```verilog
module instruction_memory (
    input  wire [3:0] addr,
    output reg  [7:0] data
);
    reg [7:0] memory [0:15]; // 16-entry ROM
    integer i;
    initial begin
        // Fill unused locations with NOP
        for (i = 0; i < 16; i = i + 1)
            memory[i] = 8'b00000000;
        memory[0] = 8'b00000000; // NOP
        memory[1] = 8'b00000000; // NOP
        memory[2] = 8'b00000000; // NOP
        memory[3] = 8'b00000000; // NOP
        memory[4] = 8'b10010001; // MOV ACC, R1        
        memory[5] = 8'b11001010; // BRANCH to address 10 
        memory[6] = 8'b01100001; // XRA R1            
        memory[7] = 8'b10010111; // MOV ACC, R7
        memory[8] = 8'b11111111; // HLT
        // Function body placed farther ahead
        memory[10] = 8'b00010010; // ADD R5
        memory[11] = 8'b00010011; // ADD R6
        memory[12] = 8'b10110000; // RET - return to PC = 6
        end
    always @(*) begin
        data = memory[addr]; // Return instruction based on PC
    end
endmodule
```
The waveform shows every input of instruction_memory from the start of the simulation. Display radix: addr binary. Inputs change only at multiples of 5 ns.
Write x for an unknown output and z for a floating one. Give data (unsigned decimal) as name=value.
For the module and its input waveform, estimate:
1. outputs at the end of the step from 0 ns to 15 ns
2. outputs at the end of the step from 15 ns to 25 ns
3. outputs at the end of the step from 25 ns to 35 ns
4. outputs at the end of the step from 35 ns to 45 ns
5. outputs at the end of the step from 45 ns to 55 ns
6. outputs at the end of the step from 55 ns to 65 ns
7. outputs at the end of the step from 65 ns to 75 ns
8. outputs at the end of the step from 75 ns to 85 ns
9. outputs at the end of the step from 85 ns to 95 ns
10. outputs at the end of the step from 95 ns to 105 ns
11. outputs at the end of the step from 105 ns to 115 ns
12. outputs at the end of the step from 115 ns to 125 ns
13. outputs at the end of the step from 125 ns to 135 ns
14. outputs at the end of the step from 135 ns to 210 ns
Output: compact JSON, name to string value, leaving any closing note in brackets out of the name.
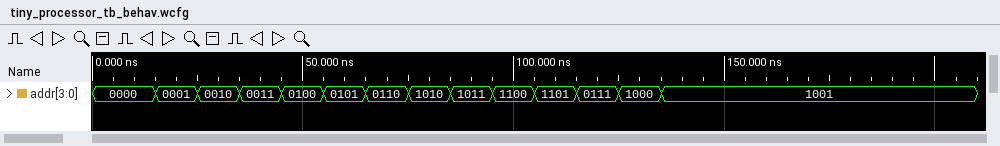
{"outputs at the end of the step from 0 ns to 15 ns": "data=0", "outputs at the end of the step from 15 ns to 25 ns": "data=0", "outputs at the end of the step from 25 ns to 35 ns": "data=0", "outputs at the end of the step from 35 ns to 45 ns": "data=0", "outputs at the end of the step from 45 ns to 55 ns": "data=145", "outputs at the end of the step from 55 ns to 65 ns": "data=202", "outputs at the end of the step from 65 ns to 75 ns": "data=97", "outputs at the end of the step from 75 ns to 85 ns": "data=18", "outputs at the end of the step from 85 ns to 95 ns": "data=19", "outputs at the end of the step from 95 ns to 105 ns": "data=176", "outputs at the end of the step from 105 ns to 115 ns": "data=0", "outputs at the end of the step from 115 ns to 125 ns": "data=151", "outputs at the end of the step from 125 ns to 135 ns": "data=255", "outputs at the end of the step from 135 ns to 210 ns": "data=0"}
